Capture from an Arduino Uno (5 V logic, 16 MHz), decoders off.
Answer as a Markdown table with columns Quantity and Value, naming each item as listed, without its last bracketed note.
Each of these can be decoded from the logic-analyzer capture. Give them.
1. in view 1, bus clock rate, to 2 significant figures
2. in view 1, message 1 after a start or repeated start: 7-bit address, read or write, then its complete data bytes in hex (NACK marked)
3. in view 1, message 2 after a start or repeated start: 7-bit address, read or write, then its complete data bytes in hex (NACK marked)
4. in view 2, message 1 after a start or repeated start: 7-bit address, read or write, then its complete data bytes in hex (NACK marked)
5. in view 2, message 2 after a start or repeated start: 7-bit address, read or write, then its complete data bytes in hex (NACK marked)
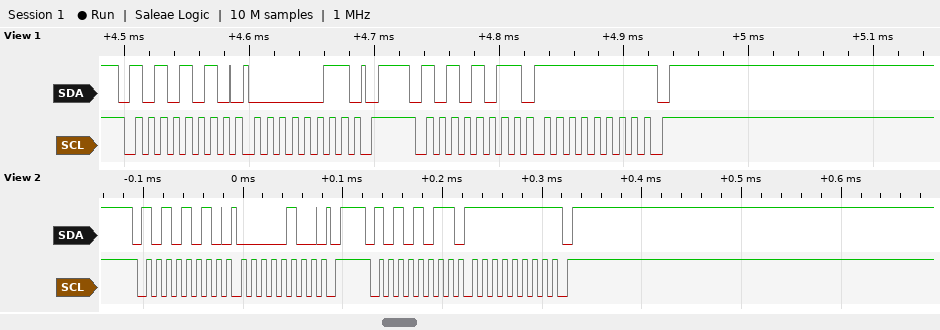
| Quantity | Value |
|---|---|
| in view 1, bus clock rate, to 2 significant figures | 100 kHz |
| in view 1, message 1 after a start or repeated start: 7-bit address, read or write, then its complete data bytes in hex | 0x55 write: 03 |
| in view 1, message 2 after a start or repeated start: 7-bit address, read or write, then its complete data bytes in hex | 0x55 read: FF NACK |
| in view 2, message 1 after a start or repeated start: 7-bit address, read or write, then its complete data bytes in hex | 0x55 write: 04 |
| in view 2, message 2 after a start or repeated start: 7-bit address, read or write, then its complete data bytes in hex | 0x55 read: FF NACK |
